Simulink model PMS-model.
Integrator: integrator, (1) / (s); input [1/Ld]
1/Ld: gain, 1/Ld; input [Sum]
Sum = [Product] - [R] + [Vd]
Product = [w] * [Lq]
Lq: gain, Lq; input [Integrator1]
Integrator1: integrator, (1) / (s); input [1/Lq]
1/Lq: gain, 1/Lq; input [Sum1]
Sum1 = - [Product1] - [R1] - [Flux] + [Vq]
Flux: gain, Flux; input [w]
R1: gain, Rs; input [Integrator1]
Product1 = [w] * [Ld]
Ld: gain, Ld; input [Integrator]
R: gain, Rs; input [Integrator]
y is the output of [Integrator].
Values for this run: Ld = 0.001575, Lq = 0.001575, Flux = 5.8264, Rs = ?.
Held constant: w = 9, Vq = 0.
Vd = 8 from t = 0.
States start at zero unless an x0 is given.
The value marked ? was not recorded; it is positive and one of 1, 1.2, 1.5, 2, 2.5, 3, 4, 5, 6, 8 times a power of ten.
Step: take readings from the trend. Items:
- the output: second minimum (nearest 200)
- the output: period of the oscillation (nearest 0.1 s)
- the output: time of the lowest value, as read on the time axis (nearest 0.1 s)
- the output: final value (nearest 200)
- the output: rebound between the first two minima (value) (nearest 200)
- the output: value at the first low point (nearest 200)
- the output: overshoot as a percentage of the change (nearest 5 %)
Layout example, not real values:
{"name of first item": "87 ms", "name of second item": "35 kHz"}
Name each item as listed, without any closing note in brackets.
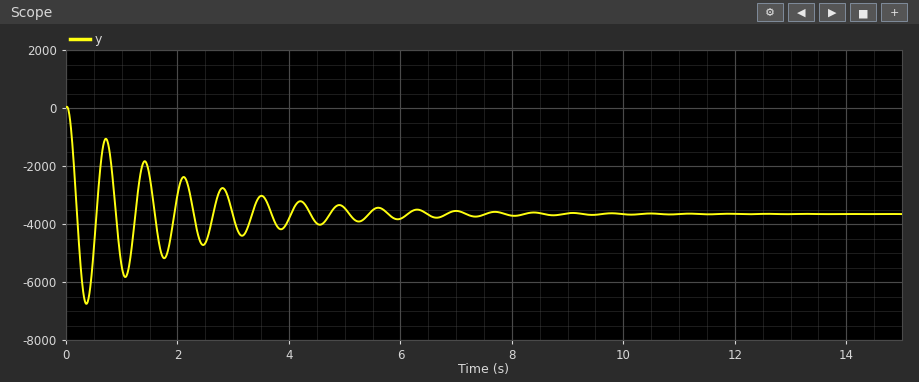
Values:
{"the output: second minimum": "-5800", "the output: period of the oscillation": "0.7 s", "the output: time of the lowest value, as read on the time axis": "0.4 s", "the output: final value": "-3600", "the output: rebound between the first two minima (value)": "-1000", "the output: value at the first low point": "-6800", "the output: overshoot as a percentage of the change": "85 %"}
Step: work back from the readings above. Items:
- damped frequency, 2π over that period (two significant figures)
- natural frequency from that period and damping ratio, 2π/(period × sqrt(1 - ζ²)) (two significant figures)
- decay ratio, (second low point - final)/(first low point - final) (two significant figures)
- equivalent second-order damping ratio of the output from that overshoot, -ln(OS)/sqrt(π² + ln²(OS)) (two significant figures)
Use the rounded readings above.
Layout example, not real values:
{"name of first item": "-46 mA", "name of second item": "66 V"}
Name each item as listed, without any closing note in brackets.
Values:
{"damped frequency, 2π over that period": "9.0 rad/s", "natural frequency from that period and damping ratio, 2π/(period × sqrt(1 - ζ²))": "9.0 rad/s", "decay ratio, (second low point - final)/(first low point - final)": "0.69", "equivalent second-order damping ratio of the output from that overshoot, -ln(OS)/sqrt(π² + ln²(OS))": "0.052"}
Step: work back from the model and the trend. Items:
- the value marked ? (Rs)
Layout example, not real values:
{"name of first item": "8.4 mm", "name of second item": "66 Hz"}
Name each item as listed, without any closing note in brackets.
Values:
{"the value marked ?": "0.0008"}
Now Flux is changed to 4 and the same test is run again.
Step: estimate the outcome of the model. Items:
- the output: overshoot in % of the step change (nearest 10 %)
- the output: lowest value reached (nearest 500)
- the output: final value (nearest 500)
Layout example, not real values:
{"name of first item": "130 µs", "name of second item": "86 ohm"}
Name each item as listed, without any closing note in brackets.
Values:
{"the output: overshoot in % of the step change": "90 %", "the output: lowest value reached": "-4500", "the output: final value": "-2500"}
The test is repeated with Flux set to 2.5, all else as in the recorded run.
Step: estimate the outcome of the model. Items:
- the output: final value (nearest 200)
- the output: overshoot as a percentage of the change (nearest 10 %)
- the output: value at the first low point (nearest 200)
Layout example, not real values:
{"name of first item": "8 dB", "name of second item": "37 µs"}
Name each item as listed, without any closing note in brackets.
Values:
{"the output: final value": "-1600", "the output: overshoot as a percentage of the change": "90 %", "the output: value at the first low point": "-3000"}
